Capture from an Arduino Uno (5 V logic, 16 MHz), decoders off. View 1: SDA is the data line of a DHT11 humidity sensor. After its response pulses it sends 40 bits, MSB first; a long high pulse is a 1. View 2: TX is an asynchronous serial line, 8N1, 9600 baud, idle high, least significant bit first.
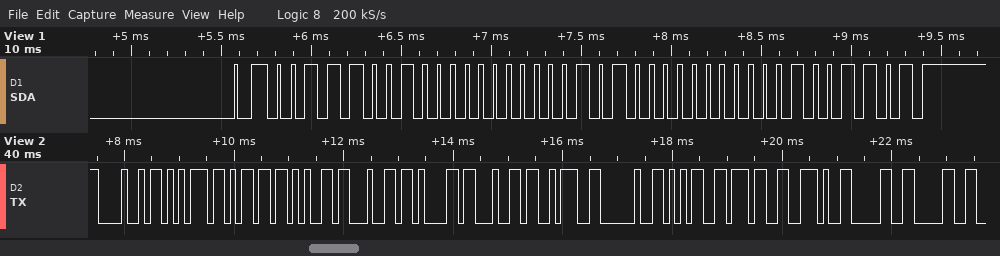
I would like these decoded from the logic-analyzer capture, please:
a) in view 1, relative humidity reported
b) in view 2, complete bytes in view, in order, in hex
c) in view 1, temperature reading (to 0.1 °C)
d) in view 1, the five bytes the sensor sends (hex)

57 %
0x48 0x75 0x6D 0x65 0x64 0x61 0x64 0x3A 0x20 0x35 0x37 0x2E 0x30 0x30
20.0 °C
39 00 14 00 4D
